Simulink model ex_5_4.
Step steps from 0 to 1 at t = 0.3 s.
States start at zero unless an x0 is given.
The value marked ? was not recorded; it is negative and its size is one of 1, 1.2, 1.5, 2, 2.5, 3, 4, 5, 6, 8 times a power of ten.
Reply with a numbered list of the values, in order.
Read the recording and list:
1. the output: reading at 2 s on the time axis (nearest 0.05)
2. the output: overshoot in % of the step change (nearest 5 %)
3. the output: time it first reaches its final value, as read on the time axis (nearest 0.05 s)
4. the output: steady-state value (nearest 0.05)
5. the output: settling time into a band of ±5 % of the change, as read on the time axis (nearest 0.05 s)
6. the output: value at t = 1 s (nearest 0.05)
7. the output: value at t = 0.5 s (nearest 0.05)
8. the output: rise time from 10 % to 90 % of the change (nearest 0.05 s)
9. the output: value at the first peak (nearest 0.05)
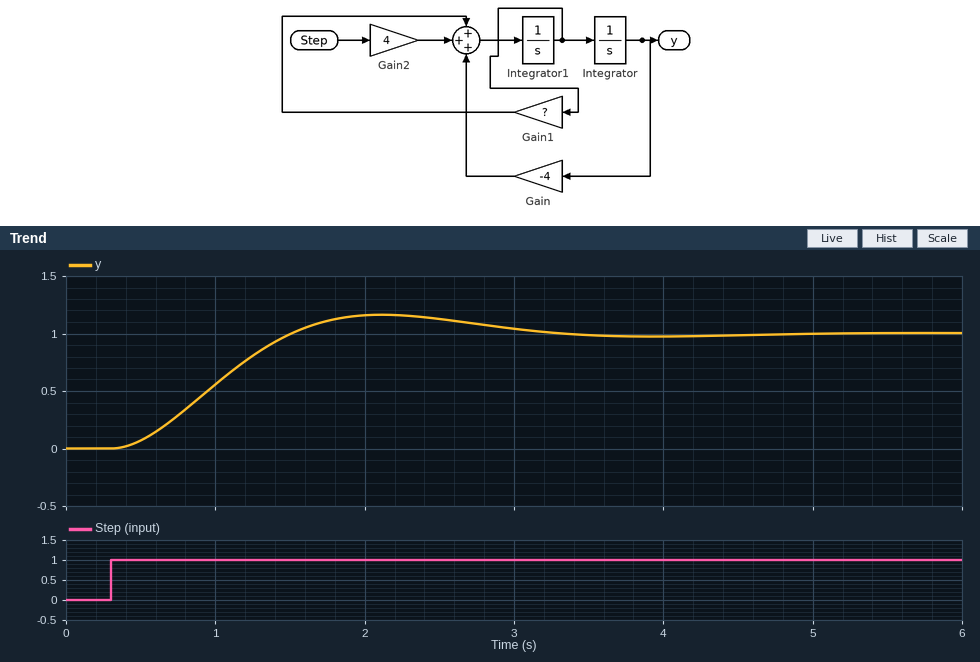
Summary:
1. 1.15
2. 15 %
3. 1.50 s
4. 1.00
5. 2.95 s
6. 0.55
7. 0.05
8. 0.80 s
9. 1.15
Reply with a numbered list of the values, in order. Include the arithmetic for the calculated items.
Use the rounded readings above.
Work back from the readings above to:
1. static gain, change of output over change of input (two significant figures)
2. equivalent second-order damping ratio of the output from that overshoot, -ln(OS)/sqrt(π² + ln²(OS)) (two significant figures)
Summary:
1. (1 - 0) / (1 - 0) = 1.0
2. ln(0.15) = -1.897; 1.897 / sqrt(9.870 + 3.599) = 0.52
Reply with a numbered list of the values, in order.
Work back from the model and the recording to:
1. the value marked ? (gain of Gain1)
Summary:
1. -2
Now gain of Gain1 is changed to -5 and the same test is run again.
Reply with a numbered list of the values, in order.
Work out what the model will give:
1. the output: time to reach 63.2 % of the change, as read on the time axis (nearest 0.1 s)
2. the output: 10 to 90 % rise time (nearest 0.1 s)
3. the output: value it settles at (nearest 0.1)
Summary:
1. 1.6 s
2. 2.3 s
3. 1.0
